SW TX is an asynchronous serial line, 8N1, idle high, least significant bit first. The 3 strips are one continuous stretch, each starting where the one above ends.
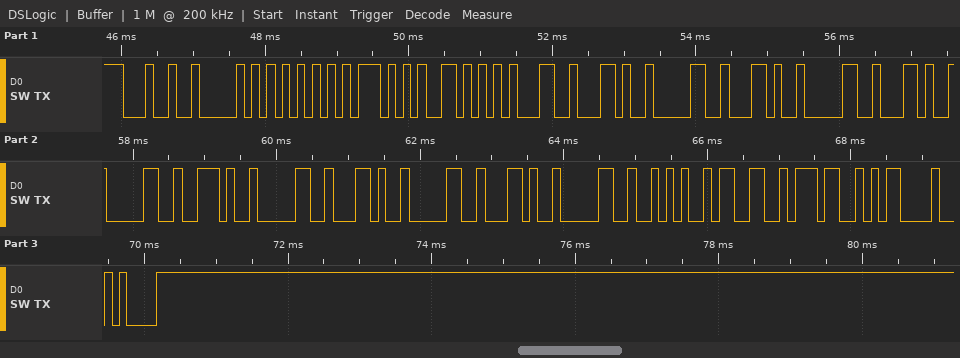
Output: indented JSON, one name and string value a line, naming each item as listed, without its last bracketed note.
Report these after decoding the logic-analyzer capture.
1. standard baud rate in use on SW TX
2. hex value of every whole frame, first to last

{
  "standard baud rate in use on SW TX": "9600 baud",
  "hex value of every whole frame, first to last": "24 50 55 57 56 31 2C 30 2C 30 2C 30 2E 30 2C 30 2C 30 2A 33 37 0D 0A"
}
